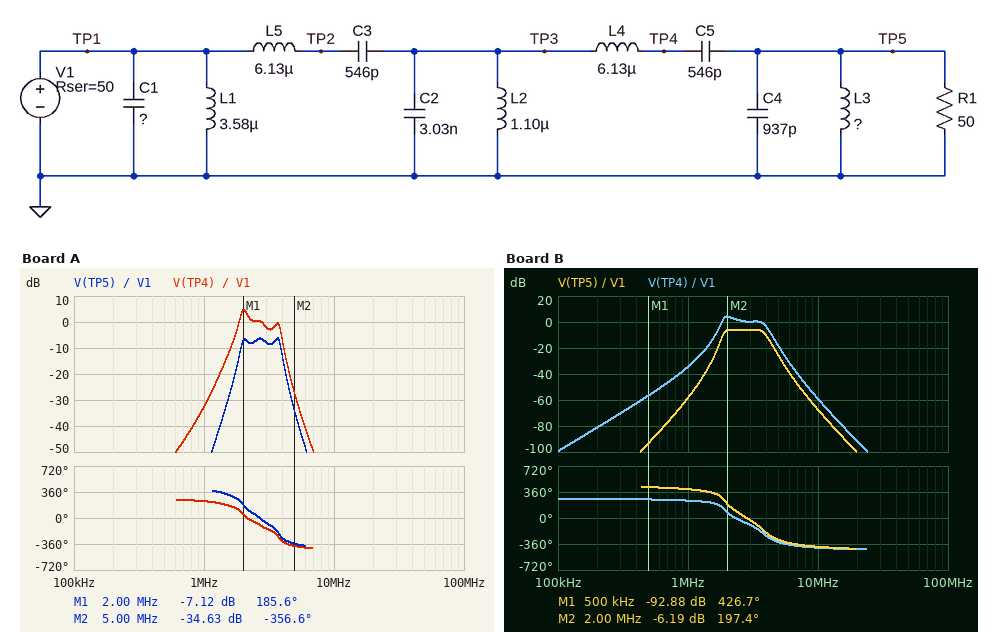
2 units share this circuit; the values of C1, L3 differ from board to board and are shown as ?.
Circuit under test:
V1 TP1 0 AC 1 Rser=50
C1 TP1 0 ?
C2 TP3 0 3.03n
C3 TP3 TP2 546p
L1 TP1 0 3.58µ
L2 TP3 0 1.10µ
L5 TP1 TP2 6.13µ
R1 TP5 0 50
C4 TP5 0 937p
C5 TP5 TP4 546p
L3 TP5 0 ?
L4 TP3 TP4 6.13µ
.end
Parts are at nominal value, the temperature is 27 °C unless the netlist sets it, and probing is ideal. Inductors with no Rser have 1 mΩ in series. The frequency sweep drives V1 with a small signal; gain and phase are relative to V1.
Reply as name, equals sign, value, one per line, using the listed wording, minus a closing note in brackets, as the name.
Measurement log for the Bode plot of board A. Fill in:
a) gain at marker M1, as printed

gain at marker M1, as printed = -7.12 dB
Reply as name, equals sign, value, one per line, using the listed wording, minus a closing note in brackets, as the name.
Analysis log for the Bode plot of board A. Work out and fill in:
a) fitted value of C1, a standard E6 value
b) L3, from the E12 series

fitted value of C1, a standard E6 value = 2.2 nF
L3, from the E12 series = 2.2 µH
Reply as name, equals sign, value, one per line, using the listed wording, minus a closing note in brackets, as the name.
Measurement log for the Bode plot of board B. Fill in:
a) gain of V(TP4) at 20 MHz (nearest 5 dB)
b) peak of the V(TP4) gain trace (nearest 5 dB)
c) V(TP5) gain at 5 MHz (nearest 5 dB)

gain of V(TP4) at 20 MHz = -90 dB
peak of the V(TP4) gain trace = 5 dB
V(TP5) gain at 5 MHz = -25 dB
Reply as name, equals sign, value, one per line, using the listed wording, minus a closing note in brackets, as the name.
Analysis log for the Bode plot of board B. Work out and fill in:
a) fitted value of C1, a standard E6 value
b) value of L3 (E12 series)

fitted value of C1, a standard E6 value = 680 pF
value of L3 = 2.7 µH
